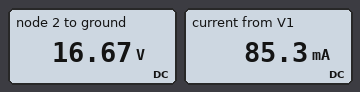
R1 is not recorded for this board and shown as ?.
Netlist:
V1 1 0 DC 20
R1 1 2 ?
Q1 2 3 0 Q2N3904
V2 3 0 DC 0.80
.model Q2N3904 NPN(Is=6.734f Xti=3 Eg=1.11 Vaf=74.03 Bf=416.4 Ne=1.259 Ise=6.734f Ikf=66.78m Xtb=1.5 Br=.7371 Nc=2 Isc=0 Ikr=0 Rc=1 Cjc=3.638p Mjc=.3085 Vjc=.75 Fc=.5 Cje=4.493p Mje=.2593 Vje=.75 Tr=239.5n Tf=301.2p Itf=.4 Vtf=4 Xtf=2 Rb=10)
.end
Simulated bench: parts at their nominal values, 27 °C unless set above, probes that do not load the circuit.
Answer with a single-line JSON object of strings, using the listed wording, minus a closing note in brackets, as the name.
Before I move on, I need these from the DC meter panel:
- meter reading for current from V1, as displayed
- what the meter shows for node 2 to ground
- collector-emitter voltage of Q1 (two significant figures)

{"meter reading for current from V1, as displayed": "85.3 mA", "what the meter shows for node 2 to ground": "16.67 V", "collector-emitter voltage of Q1": "17 V"}
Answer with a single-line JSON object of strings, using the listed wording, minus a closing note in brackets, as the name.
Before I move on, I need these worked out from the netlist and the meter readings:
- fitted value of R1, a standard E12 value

{"fitted value of R1, a standard E12 value": "39 Ω"}
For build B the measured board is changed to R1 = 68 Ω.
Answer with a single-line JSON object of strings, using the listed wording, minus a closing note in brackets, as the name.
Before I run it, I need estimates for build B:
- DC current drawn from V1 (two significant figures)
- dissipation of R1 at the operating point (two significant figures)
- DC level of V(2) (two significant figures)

{"DC current drawn from V1": "83 mA", "dissipation of R1 at the operating point": "470 mW", "DC level of V(2)": "14 V"}
